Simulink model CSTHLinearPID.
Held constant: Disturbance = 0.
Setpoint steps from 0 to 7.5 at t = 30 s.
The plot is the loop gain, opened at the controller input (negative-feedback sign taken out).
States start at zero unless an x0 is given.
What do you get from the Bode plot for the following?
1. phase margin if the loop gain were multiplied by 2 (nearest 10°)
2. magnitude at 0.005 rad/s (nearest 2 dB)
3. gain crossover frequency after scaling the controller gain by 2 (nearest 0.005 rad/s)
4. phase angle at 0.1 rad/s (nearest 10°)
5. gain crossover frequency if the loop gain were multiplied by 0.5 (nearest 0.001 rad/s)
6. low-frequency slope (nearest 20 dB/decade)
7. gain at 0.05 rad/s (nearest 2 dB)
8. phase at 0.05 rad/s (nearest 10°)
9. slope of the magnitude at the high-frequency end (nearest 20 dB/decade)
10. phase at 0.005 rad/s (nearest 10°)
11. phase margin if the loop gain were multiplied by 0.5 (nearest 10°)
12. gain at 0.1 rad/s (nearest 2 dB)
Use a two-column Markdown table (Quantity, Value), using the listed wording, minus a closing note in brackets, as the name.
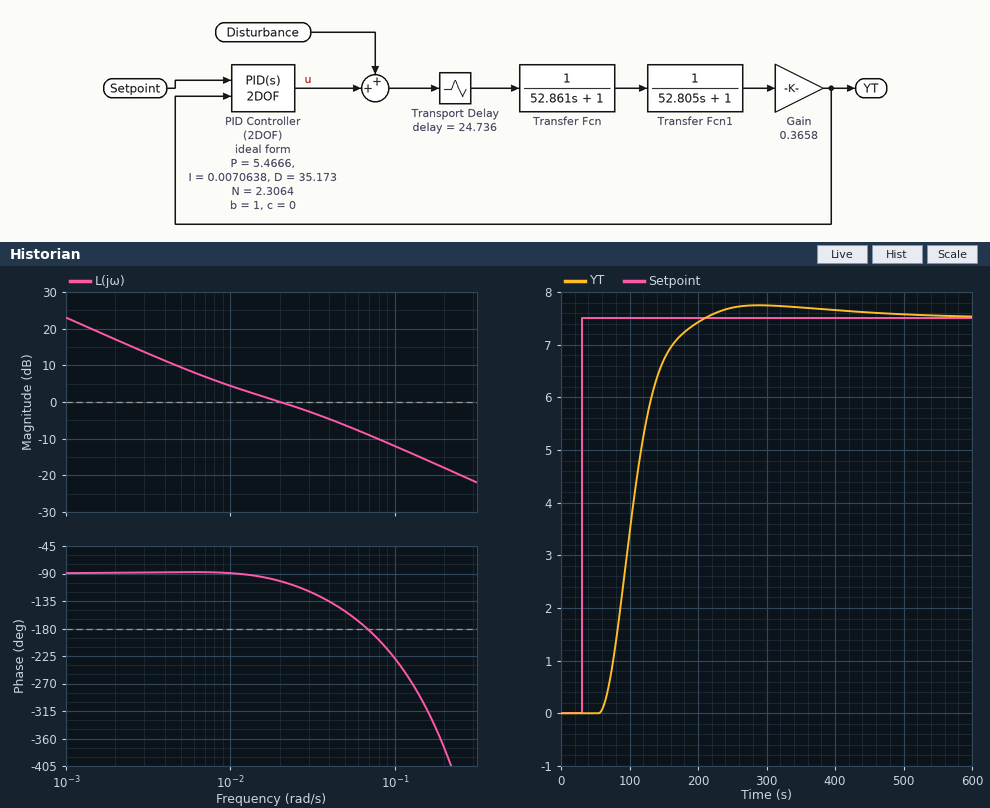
| Quantity | Value |
|---|---|
| phase margin if the loop gain were multiplied by 2 | 30° |
| magnitude at 0.005 rad/s | 10 dB |
| gain crossover frequency after scaling the controller gain by 2 | 0.050 rad/s |
| phase angle at 0.1 rad/s | -230° |
| gain crossover frequency if the loop gain were multiplied by 0.5 | 0.008 rad/s |
| low-frequency slope | -20 dB/decade |
| gain at 0.05 rad/s | -6 dB |
| phase at 0.05 rad/s | -150° |
| slope of the magnitude at the high-frequency end | -20 dB/decade |
| phase at 0.005 rad/s | -90° |
| phase margin if the loop gain were multiplied by 0.5 | 90° |
| gain at 0.1 rad/s | -12 dB |
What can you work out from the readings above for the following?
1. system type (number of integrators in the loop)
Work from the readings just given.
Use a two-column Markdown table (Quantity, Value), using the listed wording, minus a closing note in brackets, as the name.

| Quantity | Value |
|---|---|
| system type | 1 |
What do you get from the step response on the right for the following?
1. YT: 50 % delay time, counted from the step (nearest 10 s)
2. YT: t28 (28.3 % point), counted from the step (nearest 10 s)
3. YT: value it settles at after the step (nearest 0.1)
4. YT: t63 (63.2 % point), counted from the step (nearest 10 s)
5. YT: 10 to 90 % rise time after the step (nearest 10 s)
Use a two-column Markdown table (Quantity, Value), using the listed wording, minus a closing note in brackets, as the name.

| Quantity | Value |
|---|---|
| YT: 50 % delay time, counted from the step | 70 s |
| YT: t28 (28.3 % point), counted from the step | 60 s |
| YT: value it settles at after the step | 7.5 |
| YT: t63 (63.2 % point), counted from the step | 80 s |
| YT: 10 to 90 % rise time after the step | 80 s |
